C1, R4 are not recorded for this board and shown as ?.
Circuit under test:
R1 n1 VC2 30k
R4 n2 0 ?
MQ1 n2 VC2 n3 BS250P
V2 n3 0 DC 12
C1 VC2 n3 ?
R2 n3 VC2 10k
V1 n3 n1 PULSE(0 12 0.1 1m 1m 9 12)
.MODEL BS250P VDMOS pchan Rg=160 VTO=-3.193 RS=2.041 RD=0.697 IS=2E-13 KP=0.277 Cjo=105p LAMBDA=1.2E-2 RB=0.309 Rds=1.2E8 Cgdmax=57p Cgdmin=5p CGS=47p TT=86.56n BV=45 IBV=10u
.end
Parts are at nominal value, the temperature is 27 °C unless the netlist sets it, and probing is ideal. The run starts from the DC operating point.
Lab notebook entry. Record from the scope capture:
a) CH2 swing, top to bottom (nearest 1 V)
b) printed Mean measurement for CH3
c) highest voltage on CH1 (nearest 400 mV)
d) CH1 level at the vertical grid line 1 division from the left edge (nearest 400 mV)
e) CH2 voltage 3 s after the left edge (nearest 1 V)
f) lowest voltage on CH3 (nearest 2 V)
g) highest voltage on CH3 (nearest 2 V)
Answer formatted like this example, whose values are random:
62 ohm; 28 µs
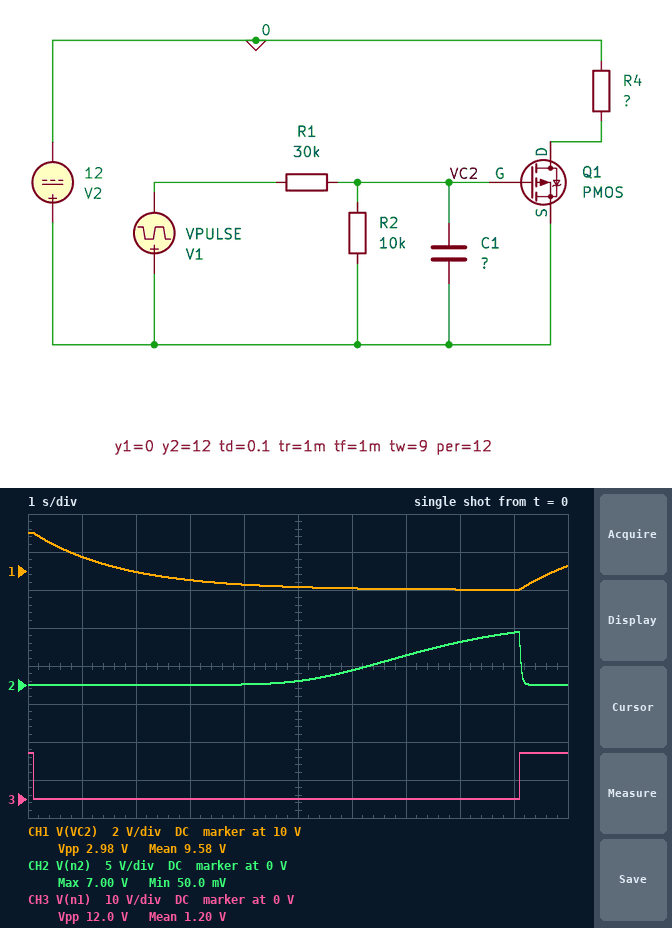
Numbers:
7 V; 1.20 V; 12.0 V; 10.8 V; 0 V; 0 V; 12 V
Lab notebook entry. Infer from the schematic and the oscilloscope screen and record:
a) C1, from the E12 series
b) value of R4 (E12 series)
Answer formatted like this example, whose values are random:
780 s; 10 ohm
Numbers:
220 µF; 330 kΩ
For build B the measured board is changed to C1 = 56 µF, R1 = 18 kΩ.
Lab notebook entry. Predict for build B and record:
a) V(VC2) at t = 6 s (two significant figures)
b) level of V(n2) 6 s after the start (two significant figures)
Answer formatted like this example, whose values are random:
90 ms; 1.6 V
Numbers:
7.7 V; 12 V
